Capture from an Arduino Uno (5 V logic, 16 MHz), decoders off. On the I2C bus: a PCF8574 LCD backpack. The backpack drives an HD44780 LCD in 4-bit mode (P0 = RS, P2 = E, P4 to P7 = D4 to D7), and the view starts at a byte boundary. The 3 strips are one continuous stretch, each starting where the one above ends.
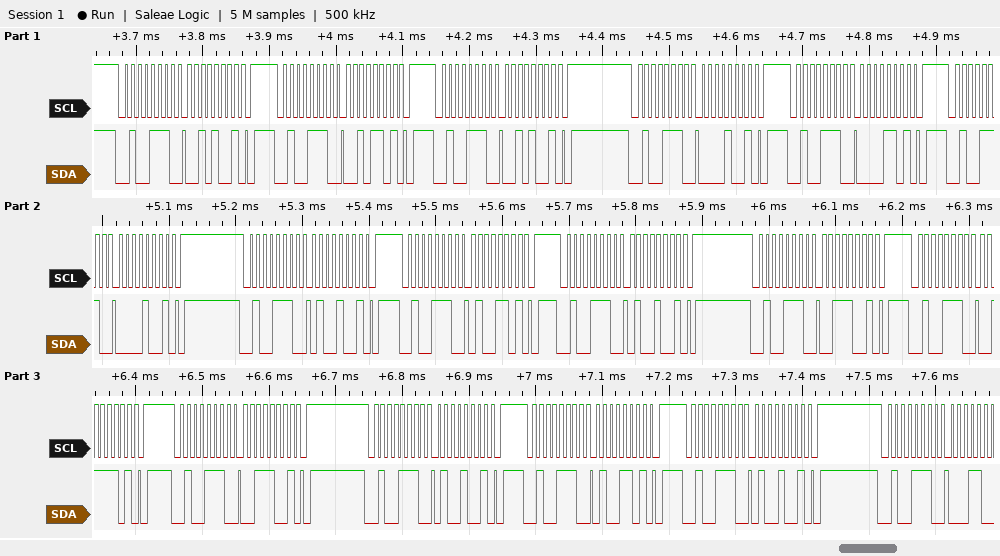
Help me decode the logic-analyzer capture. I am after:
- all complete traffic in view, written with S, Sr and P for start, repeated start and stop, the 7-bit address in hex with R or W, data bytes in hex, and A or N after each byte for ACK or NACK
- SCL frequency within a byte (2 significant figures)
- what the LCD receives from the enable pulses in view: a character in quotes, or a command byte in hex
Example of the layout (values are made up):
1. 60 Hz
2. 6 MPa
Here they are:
1. S 27W A 29 A P S 27W A 2D A P S 27W A 29 A P S 27W A 09 A P S 27W A 0D A P S 27W A 09 A P S 27W A 49 A P S 27W A 4D A P S 27W A 49 A P S 27W A 39 A P S 27W A 3D A P S 27W A 39 A P S 27W A 49 A P S 27W A 4D A P S 27W A 49 A P S 27W A
2. 100 kHz
3. ' ' 'C'
